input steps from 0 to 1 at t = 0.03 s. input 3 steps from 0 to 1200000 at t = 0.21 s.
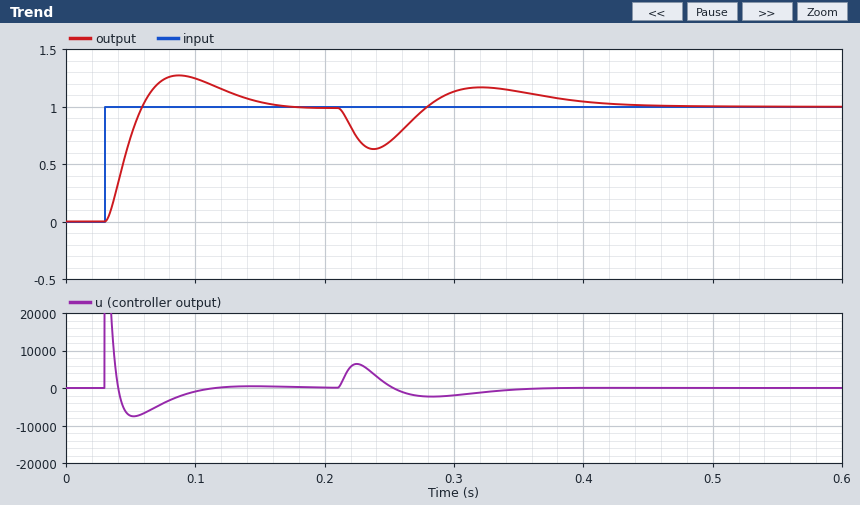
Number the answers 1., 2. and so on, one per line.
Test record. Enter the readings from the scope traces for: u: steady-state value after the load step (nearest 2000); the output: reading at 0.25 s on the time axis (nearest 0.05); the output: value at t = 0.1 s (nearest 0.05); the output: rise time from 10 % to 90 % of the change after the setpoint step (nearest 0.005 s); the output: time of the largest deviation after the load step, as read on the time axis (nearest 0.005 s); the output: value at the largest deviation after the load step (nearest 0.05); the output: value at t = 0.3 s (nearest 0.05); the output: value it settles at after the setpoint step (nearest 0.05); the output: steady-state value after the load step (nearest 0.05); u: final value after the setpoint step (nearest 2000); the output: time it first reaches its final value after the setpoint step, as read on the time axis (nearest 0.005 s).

1. 0
2. 0.70
3. 1.25
4. 0.020 s
5. 0.240 s
6. 0.65
7. 1.15
8. 1.00
9. 1.00
10. 0
11. 0.060 s
